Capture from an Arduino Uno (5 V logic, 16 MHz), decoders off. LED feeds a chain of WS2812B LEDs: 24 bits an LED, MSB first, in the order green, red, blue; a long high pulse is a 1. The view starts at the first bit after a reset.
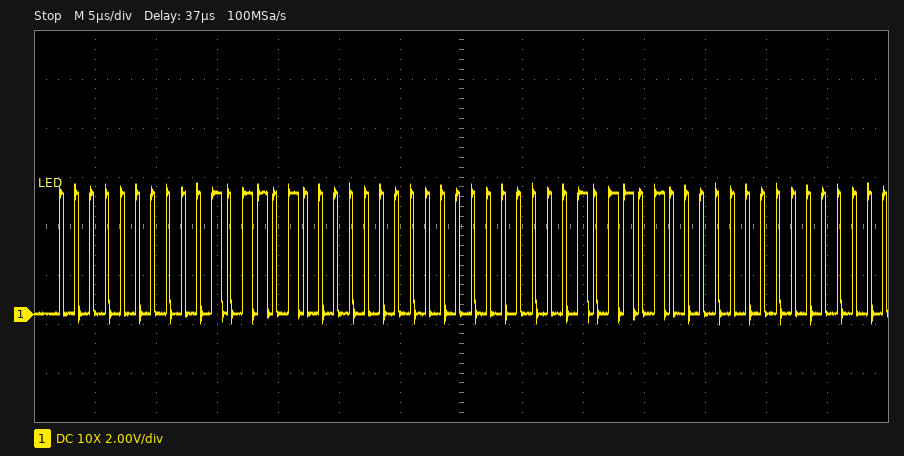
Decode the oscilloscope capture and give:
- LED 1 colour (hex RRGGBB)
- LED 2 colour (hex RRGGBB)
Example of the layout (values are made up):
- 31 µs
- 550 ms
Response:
- #2D0000
- #2D0000
